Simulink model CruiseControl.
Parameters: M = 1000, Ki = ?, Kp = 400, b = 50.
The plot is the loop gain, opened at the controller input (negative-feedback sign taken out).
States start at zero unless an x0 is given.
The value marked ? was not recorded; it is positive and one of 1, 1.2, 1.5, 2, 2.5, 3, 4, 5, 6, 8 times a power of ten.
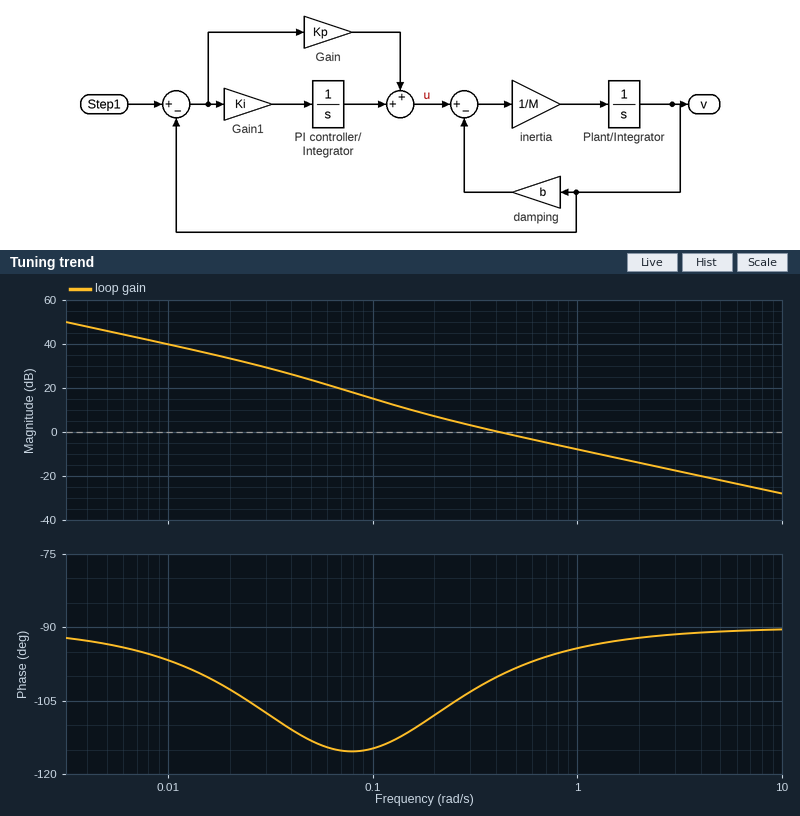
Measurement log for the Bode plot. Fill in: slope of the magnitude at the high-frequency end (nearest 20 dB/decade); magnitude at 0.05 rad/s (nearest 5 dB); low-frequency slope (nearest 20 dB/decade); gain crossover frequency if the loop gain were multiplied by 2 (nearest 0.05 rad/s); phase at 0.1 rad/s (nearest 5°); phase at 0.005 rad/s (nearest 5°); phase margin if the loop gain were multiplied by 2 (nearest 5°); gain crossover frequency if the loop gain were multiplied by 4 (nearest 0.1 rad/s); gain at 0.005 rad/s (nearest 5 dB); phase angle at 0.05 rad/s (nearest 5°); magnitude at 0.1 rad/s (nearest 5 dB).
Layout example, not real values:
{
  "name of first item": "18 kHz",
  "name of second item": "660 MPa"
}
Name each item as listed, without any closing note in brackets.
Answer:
{
  "slope of the magnitude at the high-frequency end": "-20 dB/decade",
  "magnitude at 0.05 rad/s": "25 dB",
  "low-frequency slope": "-20 dB/decade",
  "gain crossover frequency if the loop gain were multiplied by 2": "0.80 rad/s",
  "phase at 0.1 rad/s": "-115°",
  "phase at 0.005 rad/s": "-95°",
  "phase margin if the loop gain were multiplied by 2": "85°",
  "gain crossover frequency if the loop gain were multiplied by 4": "1.6 rad/s",
  "gain at 0.005 rad/s": "45 dB",
  "phase angle at 0.05 rad/s": "-115°",
  "magnitude at 0.1 rad/s": "15 dB"
}
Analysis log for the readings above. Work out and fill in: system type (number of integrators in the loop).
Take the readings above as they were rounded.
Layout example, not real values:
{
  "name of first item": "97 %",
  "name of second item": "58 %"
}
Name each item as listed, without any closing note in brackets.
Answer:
{
  "system type": "1"
}
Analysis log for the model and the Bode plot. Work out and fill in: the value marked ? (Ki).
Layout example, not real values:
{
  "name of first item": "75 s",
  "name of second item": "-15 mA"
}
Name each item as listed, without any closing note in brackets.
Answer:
{
  "the value marked ?": "50"
}
